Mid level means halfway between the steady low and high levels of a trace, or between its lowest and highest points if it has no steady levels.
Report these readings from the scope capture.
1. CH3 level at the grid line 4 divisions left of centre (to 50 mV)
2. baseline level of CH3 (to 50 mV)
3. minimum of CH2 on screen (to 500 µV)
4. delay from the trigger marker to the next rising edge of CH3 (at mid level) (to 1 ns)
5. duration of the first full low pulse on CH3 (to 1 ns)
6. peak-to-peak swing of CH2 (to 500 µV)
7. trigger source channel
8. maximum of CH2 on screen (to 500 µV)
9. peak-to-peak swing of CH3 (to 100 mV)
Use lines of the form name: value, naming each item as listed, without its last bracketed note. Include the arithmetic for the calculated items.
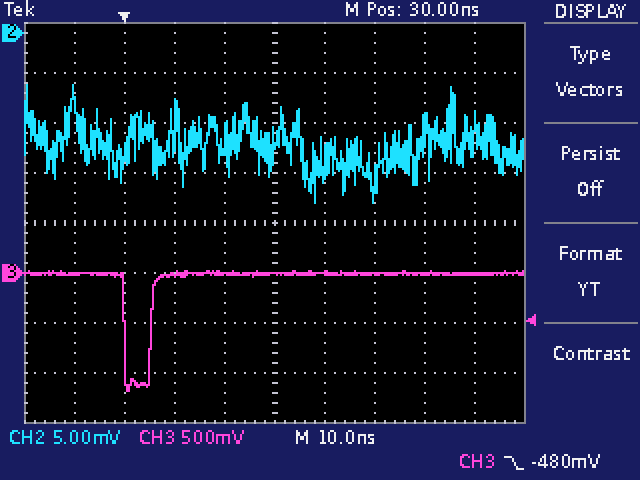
CH3 level at the grid line 4 divisions left of centre: 0 mV
baseline level of CH3: 0 mV
minimum of CH2 on screen: -17.0 mV
delay from the trigger marker to the next rising edge of CH3 (at mid level): 5 ns
duration of the first full low pulse on CH3: 5 ns
peak-to-peak swing of CH2: -5.0 mV − (-17.0 mV) = 12.0 mV
trigger source channel: CH3
maximum of CH2 on screen: -5.0 mV
peak-to-peak swing of CH3: 1.20 V
